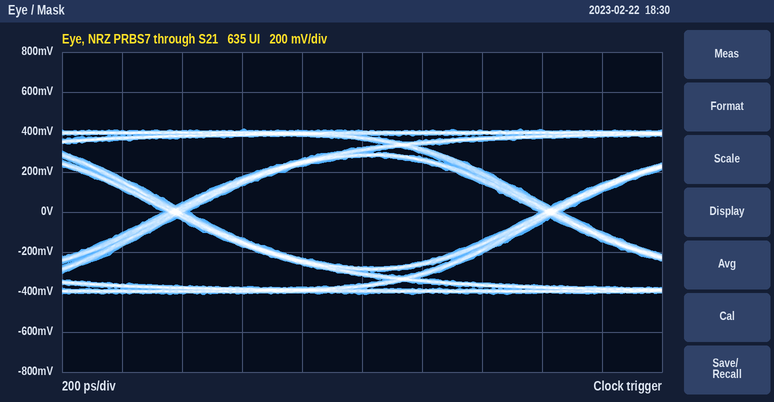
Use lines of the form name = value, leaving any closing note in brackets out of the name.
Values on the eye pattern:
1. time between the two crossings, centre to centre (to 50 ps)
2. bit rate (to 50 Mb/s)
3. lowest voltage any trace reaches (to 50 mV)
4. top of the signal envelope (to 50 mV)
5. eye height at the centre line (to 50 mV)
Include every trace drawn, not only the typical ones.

time between the two crossings, centre to centre = 1.25 ns
bit rate = 800 Mb/s
lowest voltage any trace reaches = -400 mV
top of the signal envelope = 400 mV
eye height at the centre line = 550 mV
